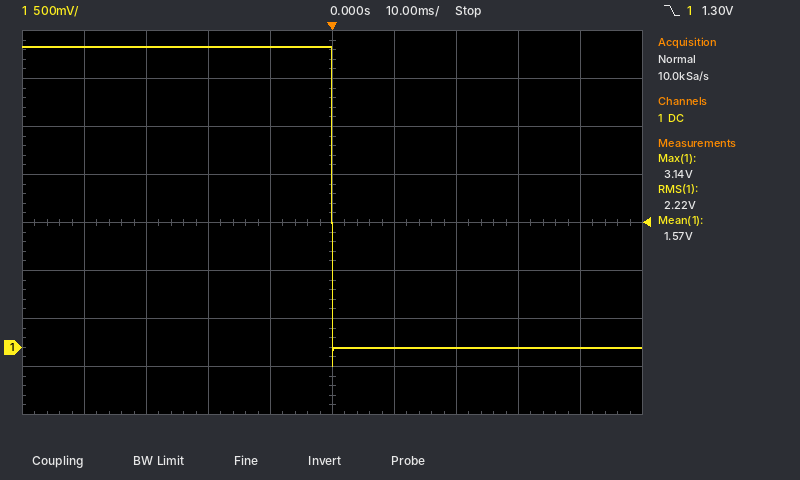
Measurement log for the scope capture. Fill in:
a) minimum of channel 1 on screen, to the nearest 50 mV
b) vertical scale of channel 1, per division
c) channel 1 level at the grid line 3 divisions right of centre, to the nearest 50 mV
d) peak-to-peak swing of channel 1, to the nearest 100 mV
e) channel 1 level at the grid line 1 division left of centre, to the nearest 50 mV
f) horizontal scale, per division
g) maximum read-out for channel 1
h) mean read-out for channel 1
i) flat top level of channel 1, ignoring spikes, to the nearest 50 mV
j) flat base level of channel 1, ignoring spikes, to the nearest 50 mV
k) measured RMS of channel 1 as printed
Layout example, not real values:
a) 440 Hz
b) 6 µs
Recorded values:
a) -200 mV
b) 500 mV
c) 0 mV
d) 3.30 V
e) 3.15 V
f) 10 ms
g) 3.14 V
h) 1.57 V
i) 3.15 V
j) 0 mV
k) 2.22 V
